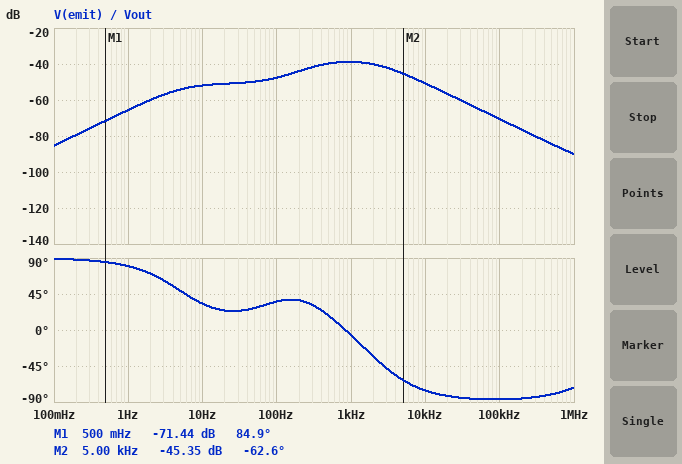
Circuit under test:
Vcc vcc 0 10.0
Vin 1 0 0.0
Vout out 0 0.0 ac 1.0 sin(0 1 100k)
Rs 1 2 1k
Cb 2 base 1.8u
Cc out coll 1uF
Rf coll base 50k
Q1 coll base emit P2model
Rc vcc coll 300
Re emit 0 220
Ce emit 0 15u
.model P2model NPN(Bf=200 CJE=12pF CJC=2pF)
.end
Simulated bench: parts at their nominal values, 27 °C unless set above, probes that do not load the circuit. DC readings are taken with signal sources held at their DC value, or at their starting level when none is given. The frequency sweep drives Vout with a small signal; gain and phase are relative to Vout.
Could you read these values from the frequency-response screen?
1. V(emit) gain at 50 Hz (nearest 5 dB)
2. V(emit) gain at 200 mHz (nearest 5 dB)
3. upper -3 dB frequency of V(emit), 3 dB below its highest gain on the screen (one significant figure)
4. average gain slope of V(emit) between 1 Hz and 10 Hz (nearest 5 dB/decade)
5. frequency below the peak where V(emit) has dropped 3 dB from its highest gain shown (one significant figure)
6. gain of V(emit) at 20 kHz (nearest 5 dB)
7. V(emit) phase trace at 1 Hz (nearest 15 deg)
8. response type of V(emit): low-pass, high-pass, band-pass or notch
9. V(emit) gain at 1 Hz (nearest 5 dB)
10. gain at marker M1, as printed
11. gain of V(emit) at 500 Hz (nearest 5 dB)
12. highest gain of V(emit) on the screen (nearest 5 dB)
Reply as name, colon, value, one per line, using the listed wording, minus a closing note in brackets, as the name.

V(emit) gain at 50 Hz: -50 dB
V(emit) gain at 200 mHz: -80 dB
upper -3 dB frequency of V(emit), 3 dB below its highest gain on the screen: 3 kHz
average gain slope of V(emit) between 1 Hz and 10 Hz: 15 dB/decade
frequency below the peak where V(emit) has dropped 3 dB from its highest gain shown: 300 Hz
gain of V(emit) at 20 kHz: -55 dB
V(emit) phase trace at 1 Hz: 75 deg
response type of V(emit): low-pass, high-pass, band-pass or notch: band-pass
V(emit) gain at 1 Hz: -65 dB
gain at marker M1, as printed: -71.44 dB
gain of V(emit) at 500 Hz: -40 dB
highest gain of V(emit) on the screen: -40 dB
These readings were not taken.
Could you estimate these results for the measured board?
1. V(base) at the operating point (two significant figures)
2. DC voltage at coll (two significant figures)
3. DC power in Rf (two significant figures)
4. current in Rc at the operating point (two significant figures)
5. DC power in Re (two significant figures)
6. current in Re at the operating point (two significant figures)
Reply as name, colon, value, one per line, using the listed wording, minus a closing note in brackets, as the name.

V(base) at the operating point: 3.5 V
DC voltage at coll: 6.4 V
DC power in Rf: 180 µW
current in Rc at the operating point: 12 mA
DC power in Re: 31 mW
current in Re at the operating point: 12 mA
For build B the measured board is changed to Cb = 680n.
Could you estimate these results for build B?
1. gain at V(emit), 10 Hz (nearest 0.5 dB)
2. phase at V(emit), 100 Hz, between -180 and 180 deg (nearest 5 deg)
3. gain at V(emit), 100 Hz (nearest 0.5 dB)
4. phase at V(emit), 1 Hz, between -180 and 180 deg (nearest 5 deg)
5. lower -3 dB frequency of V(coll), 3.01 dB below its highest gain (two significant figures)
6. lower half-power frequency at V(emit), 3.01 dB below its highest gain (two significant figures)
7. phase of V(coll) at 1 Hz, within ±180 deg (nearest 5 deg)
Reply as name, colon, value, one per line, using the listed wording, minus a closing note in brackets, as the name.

gain at V(emit), 10 Hz: -47.5 dB
phase at V(emit), 100 Hz, between -180 and 180 deg: 15 deg
gain at V(emit), 100 Hz: -43.0 dB
phase at V(emit), 1 Hz, between -180 and 180 deg: 85 deg
lower -3 dB frequency of V(coll), 3.01 dB below its highest gain: 850 Hz
lower half-power frequency at V(emit), 3.01 dB below its highest gain: 190 Hz
phase of V(coll) at 1 Hz, within ±180 deg: 90 deg
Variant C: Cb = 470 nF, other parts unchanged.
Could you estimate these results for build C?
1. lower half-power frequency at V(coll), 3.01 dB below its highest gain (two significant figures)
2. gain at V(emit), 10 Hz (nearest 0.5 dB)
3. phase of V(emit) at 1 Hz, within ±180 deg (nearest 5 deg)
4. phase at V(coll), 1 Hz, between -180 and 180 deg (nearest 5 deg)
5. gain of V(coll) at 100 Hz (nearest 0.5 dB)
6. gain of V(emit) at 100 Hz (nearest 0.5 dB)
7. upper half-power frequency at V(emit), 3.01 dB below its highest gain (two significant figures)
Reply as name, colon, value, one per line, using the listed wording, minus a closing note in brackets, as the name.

lower half-power frequency at V(coll), 3.01 dB below its highest gain: 850 Hz
gain at V(emit), 10 Hz: -46.5 dB
phase of V(emit) at 1 Hz, within ±180 deg: 85 deg
phase at V(coll), 1 Hz, between -180 and 180 deg: 90 deg
gain of V(coll) at 100 Hz: -16.0 dB
gain of V(emit) at 100 Hz: -41.0 dB
upper half-power frequency at V(emit), 3.01 dB below its highest gain: 2.8 kHz
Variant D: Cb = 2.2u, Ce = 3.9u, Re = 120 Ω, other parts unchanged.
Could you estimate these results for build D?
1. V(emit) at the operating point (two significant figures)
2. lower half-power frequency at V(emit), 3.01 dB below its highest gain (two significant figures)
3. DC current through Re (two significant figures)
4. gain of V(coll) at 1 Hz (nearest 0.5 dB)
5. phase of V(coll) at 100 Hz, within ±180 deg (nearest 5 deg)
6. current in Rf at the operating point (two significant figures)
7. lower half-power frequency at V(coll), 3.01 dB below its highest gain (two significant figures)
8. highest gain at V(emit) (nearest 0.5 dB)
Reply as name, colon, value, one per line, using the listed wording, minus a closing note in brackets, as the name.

V(emit) at the operating point: 1.6 V
lower half-power frequency at V(emit), 3.01 dB below its highest gain: 450 Hz
DC current through Re: 14 mA
gain of V(coll) at 1 Hz: -59.5 dB
phase of V(coll) at 100 Hz, within ±180 deg: 80 deg
current in Rf at the operating point: 68 µA
lower half-power frequency at V(coll), 3.01 dB below its highest gain: 610 Hz
highest gain at V(emit): -36.0 dB
